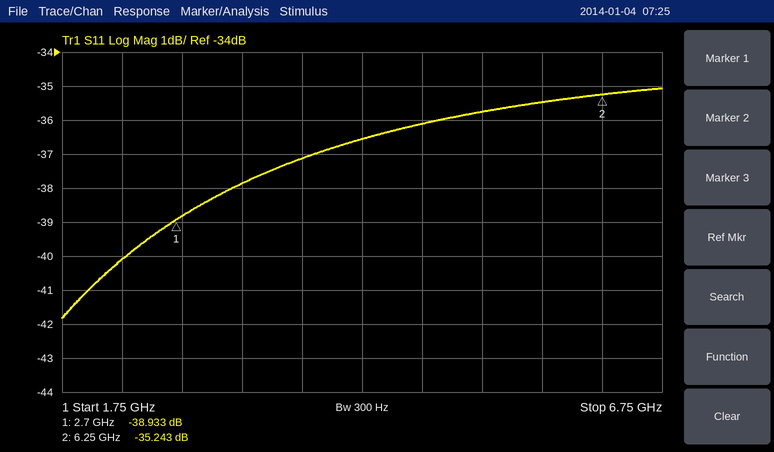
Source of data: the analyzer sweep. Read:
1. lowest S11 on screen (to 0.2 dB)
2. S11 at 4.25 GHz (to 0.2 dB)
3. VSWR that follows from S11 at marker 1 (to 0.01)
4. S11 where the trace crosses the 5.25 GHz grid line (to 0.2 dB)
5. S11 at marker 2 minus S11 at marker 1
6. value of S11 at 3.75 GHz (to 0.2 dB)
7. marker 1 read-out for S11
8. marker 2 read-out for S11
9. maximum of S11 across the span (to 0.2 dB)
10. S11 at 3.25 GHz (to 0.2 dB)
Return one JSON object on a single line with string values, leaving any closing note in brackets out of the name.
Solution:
{"lowest S11 on screen": "-41.8 dB", "S11 at 4.25 GHz": "-36.6 dB", "VSWR that follows from S11 at marker 1": "1.02", "S11 where the trace crosses the 5.25 GHz grid line": "-35.8 dB", "S11 at marker 2 minus S11 at marker 1": "3.690 dB", "value of S11 at 3.75 GHz": "-37.2 dB", "marker 1 read-out for S11": "-38.933 dB", "marker 2 read-out for S11": "-35.243 dB", "maximum of S11 across the span": "-35.0 dB", "S11 at 3.25 GHz": "-37.8 dB"}
